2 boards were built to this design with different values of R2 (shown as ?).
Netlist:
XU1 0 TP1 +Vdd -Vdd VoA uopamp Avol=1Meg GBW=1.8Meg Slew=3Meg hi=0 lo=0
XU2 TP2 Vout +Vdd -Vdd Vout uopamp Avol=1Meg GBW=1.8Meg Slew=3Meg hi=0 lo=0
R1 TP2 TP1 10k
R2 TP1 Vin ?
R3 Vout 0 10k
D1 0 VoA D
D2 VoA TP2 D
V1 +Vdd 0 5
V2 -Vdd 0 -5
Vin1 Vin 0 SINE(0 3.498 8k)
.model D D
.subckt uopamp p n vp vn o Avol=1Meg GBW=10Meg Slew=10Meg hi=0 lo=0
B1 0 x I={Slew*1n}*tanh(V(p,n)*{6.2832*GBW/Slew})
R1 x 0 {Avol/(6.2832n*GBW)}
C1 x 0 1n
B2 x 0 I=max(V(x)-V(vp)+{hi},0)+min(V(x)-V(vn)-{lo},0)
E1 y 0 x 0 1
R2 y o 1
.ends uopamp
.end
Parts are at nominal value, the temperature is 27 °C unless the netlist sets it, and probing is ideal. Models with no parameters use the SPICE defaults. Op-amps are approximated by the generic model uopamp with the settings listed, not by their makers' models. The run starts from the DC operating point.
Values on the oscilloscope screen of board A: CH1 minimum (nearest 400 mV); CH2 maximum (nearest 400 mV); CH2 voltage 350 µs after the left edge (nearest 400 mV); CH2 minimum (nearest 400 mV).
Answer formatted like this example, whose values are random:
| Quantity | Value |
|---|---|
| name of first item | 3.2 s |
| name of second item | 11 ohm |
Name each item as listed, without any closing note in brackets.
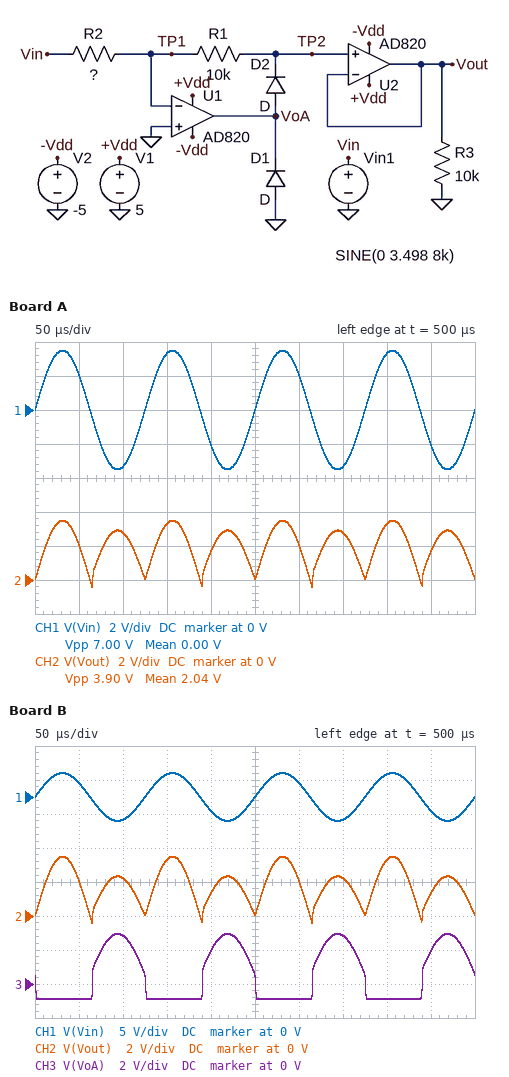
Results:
| Quantity | Value |
|---|---|
| CH1 minimum | -3.6 V |
| CH2 maximum | 3.6 V |
| CH2 voltage 350 µs after the left edge | 2.8 V |
| CH2 minimum | -400 mV |
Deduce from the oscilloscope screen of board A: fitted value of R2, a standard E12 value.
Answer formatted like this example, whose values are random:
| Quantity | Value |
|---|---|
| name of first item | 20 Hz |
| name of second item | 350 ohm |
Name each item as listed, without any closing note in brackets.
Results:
| Quantity | Value |
|---|---|
| fitted value of R2, a standard E12 value | 12 kΩ |
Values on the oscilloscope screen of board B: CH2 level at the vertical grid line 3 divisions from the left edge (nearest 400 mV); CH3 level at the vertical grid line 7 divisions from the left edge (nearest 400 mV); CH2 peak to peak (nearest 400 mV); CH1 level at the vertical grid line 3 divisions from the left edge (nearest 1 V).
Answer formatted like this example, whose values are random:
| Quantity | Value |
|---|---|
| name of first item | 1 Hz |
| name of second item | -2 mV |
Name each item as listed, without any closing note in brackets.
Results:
| Quantity | Value |
|---|---|
| CH2 level at the vertical grid line 3 divisions from the left edge | 3.2 V |
| CH3 level at the vertical grid line 7 divisions from the left edge | 2.8 V |
| CH2 peak to peak | 4.0 V |
| CH1 level at the vertical grid line 3 divisions from the left edge | 3 V |
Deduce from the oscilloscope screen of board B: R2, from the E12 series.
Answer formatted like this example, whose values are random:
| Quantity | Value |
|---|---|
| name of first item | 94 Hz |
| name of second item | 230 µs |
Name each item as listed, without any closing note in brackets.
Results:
| Quantity | Value |
|---|---|
| R2, from the E12 series | 15 kΩ |
